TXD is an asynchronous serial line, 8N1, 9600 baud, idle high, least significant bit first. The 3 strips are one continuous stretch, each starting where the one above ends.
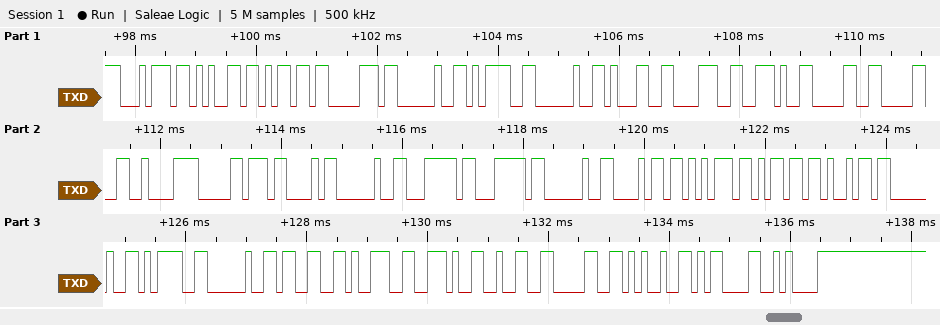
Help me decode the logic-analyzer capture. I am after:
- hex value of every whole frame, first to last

74 65 6D 70 20 3D 20 31 38 2E 30 30 C2 B0 43 20 7C 7C 20 68 75 6D 69 20 3D 20 33 39 2E 32 30 25 0D 0A
